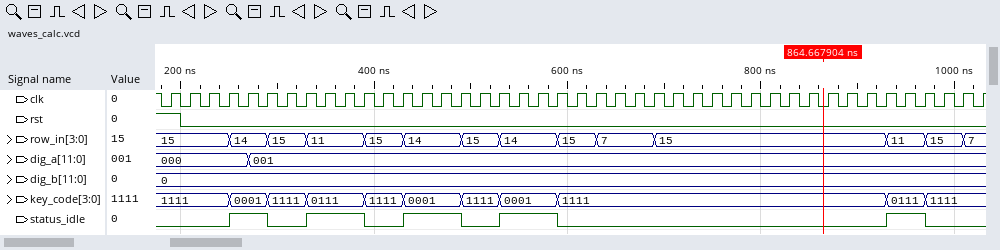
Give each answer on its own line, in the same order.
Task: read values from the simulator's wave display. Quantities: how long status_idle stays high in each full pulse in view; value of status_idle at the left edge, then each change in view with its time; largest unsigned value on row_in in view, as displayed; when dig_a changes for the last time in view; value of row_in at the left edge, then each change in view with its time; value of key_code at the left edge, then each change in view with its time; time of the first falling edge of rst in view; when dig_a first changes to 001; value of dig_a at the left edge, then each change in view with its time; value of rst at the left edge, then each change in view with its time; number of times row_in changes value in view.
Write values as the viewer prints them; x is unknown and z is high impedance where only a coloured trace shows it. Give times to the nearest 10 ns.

40 ns, 60 ns, 60 ns, 60 ns, 40 ns
0, 1 at 250 ns, 0 at 290 ns, 1 at 330 ns, 0 at 390 ns, 1 at 430 ns, 0 at 490 ns, 1 at 530 ns, 0 at 590 ns, 1 at 930 ns, 0 at 970 ns
15
270 ns
15, 14 at 250 ns, 15 at 290 ns, 11 at 330 ns, 15 at 390 ns, 14 at 430 ns, 15 at 490 ns, 14 at 530 ns, 15 at 590 ns, 7 at 630 ns, 15 at 690 ns, 11 at 930 ns, 15 at 970 ns, 7 at 1010 ns
1111, 0001 at 250 ns, 1111 at 290 ns, 0111 at 330 ns, 1111 at 390 ns, 0001 at 430 ns, 1111 at 490 ns, 0001 at 530 ns, 1111 at 590 ns, 0111 at 930 ns, 1111 at 970 ns
200 ns
270 ns
000, 001 at 270 ns
1, 0 at 200 ns
13
